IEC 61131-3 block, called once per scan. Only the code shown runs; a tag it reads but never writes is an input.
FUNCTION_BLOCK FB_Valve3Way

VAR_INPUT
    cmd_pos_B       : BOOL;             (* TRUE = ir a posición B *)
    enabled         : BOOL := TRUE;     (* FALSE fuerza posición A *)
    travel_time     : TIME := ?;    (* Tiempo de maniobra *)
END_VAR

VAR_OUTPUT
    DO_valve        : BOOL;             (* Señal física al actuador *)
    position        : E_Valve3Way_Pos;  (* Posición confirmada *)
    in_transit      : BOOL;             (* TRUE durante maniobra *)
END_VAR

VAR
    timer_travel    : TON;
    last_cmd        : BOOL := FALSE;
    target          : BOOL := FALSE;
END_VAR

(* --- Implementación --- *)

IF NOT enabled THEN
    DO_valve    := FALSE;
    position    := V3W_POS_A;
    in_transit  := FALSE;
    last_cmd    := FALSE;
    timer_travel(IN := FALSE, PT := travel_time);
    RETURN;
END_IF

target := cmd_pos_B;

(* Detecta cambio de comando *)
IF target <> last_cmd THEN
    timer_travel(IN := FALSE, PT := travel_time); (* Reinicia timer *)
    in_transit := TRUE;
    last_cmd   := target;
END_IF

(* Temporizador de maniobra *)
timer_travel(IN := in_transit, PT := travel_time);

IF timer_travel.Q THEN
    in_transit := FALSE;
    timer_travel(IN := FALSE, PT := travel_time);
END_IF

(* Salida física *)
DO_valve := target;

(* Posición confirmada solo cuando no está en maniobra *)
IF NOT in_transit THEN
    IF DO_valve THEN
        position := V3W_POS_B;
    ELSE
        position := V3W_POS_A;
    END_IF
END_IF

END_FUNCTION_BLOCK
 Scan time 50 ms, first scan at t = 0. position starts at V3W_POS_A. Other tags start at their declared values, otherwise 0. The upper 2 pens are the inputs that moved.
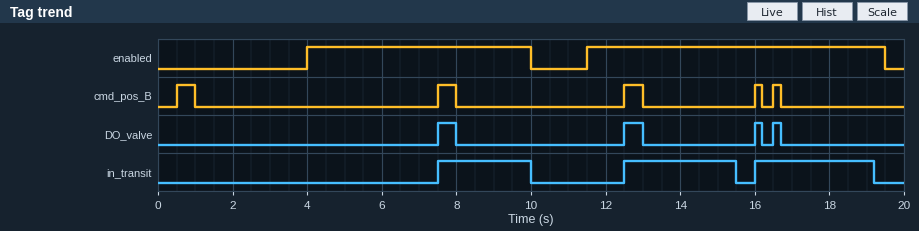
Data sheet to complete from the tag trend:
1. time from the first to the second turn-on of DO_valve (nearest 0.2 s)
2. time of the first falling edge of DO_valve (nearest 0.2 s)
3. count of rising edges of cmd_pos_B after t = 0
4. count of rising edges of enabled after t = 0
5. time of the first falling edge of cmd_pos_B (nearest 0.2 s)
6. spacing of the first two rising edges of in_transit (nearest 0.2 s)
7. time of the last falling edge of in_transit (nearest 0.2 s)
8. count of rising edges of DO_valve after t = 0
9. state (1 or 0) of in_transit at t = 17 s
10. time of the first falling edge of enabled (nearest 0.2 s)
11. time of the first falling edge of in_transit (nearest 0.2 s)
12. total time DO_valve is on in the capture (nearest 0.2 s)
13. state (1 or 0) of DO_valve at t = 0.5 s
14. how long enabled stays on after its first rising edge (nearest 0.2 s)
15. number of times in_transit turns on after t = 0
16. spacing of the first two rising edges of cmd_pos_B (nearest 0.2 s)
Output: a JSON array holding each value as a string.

["5.0 s", "8.0 s", "5", "2", "1.0 s", "5.0 s", "19.2 s", "4", "1", "10.0 s", "10.0 s", "1.4 s", "0", "6.0 s", "3", "7.0 s"]
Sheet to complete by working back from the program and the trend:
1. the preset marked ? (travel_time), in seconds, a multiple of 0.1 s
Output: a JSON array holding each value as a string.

["2.5 s"]
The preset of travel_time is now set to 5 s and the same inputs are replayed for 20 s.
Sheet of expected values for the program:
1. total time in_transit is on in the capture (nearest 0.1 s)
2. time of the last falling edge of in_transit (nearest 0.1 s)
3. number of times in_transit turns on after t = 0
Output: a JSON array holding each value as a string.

["9.5 s", "19.5 s", "2"]
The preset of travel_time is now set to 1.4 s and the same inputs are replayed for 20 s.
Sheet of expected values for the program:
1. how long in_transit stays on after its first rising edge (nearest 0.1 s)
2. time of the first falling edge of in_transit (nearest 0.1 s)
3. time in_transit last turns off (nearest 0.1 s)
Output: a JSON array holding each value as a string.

["1.9 s", "9.4 s", "18.1 s"]
